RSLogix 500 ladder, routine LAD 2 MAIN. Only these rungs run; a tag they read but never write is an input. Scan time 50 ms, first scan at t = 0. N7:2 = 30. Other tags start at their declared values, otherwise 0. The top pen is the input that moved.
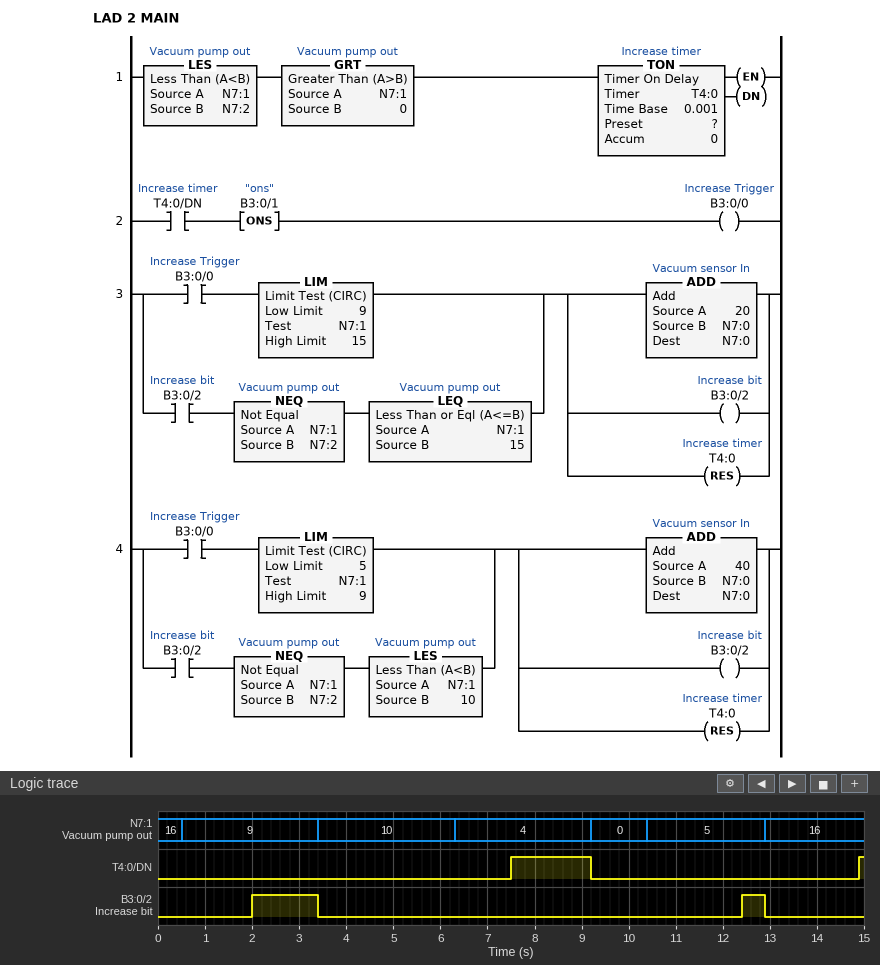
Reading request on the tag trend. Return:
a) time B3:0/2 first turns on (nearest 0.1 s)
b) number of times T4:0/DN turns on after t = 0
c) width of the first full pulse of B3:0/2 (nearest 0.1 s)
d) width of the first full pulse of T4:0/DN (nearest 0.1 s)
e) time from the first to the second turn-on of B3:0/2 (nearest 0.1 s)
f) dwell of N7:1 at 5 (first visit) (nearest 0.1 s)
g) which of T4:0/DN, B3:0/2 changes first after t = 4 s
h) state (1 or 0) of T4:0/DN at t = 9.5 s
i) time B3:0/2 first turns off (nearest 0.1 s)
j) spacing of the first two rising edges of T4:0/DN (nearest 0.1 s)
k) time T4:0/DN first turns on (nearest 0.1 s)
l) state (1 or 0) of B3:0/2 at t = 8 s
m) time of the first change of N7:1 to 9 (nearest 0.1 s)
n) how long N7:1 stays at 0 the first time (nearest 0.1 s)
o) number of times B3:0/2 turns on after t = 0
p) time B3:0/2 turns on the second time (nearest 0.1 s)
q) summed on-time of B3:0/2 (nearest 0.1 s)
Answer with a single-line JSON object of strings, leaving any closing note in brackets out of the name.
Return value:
{"time B3:0/2 first turns on": "2.0 s", "number of times T4:0/DN turns on after t = 0": "2", "width of the first full pulse of B3:0/2": "1.4 s", "width of the first full pulse of T4:0/DN": "1.7 s", "time from the first to the second turn-on of B3:0/2": "10.4 s", "dwell of N7:1 at 5 (first visit)": "2.5 s", "which of T4:0/DN, B3:0/2 changes first after t = 4 s": "T4:0/DN", "state (1 or 0) of T4:0/DN at t = 9.5 s": "0", "time B3:0/2 first turns off": "3.4 s", "spacing of the first two rising edges of T4:0/DN": "7.4 s", "time T4:0/DN first turns on": "7.5 s", "state (1 or 0) of B3:0/2 at t = 8 s": "0", "time of the first change of N7:1 to 9": "0.5 s", "how long N7:1 stays at 0 the first time": "1.2 s", "number of times B3:0/2 turns on after t = 0": "2", "time B3:0/2 turns on the second time": "12.4 s", "summed on-time of B3:0/2": "1.9 s"}
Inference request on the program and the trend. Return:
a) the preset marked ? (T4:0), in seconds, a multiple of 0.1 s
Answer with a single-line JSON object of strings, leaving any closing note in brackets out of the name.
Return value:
{"the preset marked ? (T4:0), in seconds, a multiple of 0.1 s": "2.0 s"}
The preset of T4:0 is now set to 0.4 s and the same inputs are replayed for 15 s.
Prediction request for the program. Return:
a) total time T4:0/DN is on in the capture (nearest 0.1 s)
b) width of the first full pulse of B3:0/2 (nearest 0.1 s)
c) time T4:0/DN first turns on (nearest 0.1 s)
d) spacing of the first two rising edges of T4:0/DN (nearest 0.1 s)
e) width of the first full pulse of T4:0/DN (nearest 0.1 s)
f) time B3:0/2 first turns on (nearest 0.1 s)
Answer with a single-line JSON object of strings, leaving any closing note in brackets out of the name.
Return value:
{"total time T4:0/DN is on in the capture": "10.5 s", "width of the first full pulse of B3:0/2": "2.1 s", "time T4:0/DN first turns on": "0.4 s", "spacing of the first two rising edges of T4:0/DN": "12.9 s", "width of the first full pulse of T4:0/DN": "8.8 s", "time B3:0/2 first turns on": "10.8 s"}
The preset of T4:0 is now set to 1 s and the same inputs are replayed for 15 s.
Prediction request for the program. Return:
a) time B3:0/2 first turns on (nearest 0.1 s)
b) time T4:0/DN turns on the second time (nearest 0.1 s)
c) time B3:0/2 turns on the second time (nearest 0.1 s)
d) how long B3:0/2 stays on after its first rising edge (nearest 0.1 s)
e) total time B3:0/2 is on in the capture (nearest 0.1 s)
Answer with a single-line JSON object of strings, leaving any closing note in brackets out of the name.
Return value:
{"time B3:0/2 first turns on": "1.0 s", "time T4:0/DN turns on the second time": "13.9 s", "time B3:0/2 turns on the second time": "11.4 s", "how long B3:0/2 stays on after its first rising edge": "2.4 s", "total time B3:0/2 is on in the capture": "3.9 s"}
